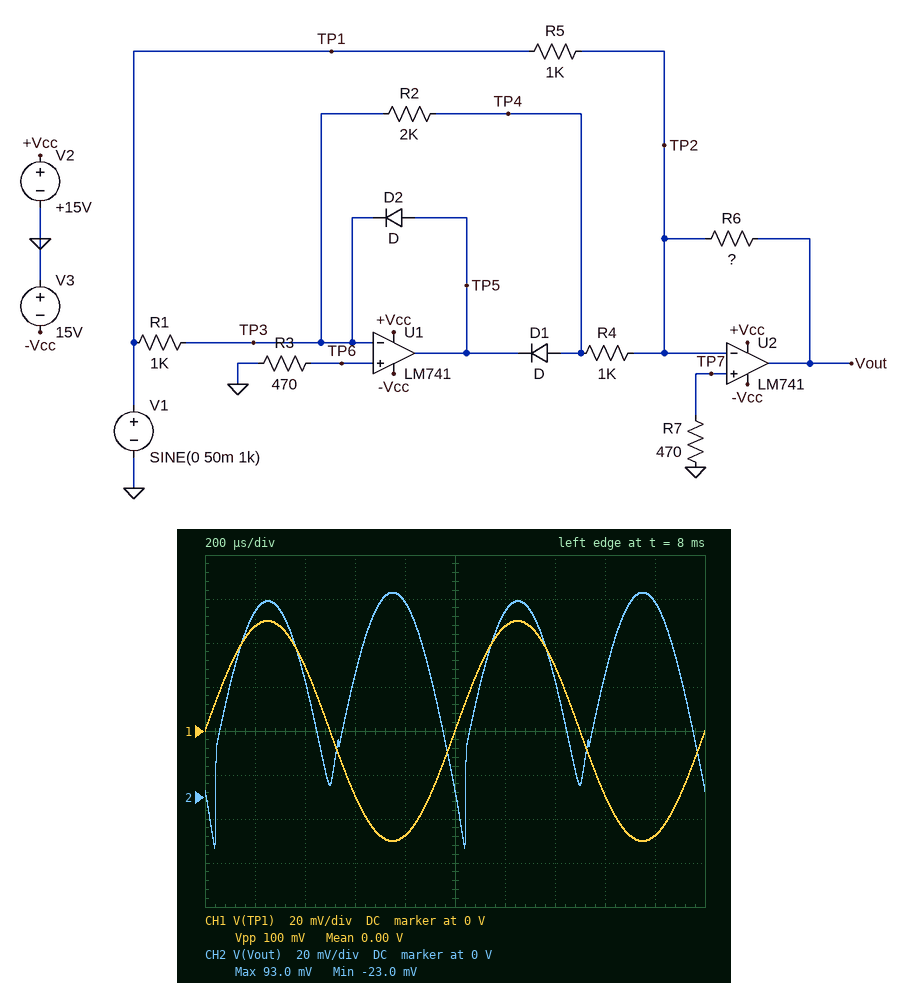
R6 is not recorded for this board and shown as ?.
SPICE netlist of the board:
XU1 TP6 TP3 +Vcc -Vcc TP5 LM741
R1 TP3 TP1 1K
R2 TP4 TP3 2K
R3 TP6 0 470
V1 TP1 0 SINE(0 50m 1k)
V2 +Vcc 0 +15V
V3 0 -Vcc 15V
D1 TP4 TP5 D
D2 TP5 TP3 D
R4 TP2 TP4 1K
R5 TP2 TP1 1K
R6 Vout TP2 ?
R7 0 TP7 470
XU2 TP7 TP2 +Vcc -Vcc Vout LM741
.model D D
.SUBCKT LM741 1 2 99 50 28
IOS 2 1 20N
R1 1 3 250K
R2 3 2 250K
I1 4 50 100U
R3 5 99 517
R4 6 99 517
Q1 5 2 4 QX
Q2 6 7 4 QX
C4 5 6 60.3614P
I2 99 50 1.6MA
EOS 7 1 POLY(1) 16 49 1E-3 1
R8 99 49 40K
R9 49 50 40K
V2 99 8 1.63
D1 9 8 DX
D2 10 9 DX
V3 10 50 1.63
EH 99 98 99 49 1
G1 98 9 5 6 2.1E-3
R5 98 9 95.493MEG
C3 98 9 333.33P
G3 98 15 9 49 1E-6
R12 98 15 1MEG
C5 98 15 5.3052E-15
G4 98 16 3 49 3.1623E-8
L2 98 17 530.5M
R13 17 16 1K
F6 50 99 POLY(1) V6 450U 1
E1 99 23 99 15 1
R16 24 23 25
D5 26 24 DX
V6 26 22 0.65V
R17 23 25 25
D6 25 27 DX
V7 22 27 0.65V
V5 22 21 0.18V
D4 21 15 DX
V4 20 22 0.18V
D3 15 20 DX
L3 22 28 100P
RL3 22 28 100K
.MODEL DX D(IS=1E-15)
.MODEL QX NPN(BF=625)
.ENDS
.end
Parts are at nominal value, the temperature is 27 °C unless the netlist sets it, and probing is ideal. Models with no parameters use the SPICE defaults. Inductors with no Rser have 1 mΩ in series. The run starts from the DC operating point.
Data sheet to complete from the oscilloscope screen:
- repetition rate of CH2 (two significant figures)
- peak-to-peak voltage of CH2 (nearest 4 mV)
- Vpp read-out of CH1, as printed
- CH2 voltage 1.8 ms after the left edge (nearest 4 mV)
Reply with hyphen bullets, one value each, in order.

- 2.0 kHz
- 116 mV
- 100 mV
- 88 mV
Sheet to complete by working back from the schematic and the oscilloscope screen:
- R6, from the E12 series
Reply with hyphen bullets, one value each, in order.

- 1.8 kΩ
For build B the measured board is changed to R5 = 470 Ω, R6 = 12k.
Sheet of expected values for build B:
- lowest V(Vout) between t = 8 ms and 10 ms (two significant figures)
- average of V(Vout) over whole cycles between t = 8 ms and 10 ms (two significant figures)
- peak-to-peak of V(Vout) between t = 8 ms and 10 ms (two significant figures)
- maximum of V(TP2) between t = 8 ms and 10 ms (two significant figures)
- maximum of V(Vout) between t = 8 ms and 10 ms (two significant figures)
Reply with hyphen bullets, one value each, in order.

- -270 mV
- 390 mV
- 1.6 V
- 2.4 mV
- 1.3 V
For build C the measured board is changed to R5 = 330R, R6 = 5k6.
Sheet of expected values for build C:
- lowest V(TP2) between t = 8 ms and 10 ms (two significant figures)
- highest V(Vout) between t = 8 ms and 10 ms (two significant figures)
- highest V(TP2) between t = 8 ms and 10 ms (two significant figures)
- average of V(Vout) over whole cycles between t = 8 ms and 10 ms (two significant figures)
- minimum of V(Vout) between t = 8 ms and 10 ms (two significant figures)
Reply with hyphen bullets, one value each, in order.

- -1.8 mV
- 870 mV
- 1.9 mV
- 190 mV
- -280 mV
